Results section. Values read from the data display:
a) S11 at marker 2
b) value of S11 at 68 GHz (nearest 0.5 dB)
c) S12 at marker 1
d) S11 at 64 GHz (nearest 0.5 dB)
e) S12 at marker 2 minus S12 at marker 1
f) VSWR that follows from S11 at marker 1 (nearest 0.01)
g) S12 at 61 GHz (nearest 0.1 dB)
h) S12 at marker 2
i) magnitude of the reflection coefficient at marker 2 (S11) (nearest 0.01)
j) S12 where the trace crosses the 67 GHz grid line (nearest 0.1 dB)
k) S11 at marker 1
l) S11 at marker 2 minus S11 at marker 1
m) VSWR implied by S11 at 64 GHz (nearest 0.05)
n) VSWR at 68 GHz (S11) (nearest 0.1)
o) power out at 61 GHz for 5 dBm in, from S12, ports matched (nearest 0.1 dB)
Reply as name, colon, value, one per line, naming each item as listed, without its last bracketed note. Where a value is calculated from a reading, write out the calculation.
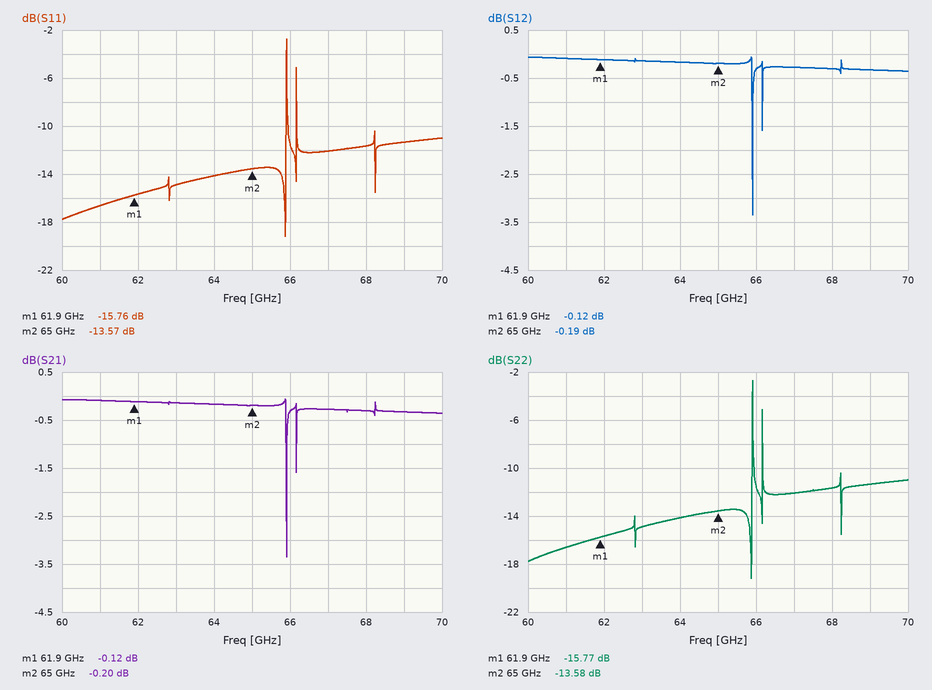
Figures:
S11 at marker 2: -13.57 dB
value of S11 at 68 GHz: -11.5 dB
S12 at marker 1: -0.12 dB
S11 at 64 GHz: -14.0 dB
S12 at marker 2 minus S12 at marker 1: -0.19 − (-0.12) = -0.07 dB
VSWR that follows from S11 at marker 1: (1 + 0.1629)/(1 − 0.1629) ≈ 1.39
S12 at 61 GHz: -0.1 dB
S12 at marker 2: -0.19 dB
magnitude of the reflection coefficient at marker 2 (S11): 10^(-13.57/20) ≈ 0.21
S12 where the trace crosses the 67 GHz grid line: -0.3 dB
S11 at marker 1: -15.76 dB
S11 at marker 2 minus S11 at marker 1: -13.57 − (-15.76) = 2.19 dB
VSWR implied by S11 at 64 GHz: |Γ| = 10^(-14/20) = 0.1995; VSWR = (1 + 0.1995)/(1 − 0.1995) ≈ 1.50
VSWR at 68 GHz (S11): |Γ| = 10^(-11.5/20) = 0.2661; VSWR = (1 + 0.2661)/(1 − 0.2661) ≈ 1.7
power out at 61 GHz for 5 dBm in, from S12, ports matched: 5 dBm + (-0.1 dB) = 4.9 dBm
